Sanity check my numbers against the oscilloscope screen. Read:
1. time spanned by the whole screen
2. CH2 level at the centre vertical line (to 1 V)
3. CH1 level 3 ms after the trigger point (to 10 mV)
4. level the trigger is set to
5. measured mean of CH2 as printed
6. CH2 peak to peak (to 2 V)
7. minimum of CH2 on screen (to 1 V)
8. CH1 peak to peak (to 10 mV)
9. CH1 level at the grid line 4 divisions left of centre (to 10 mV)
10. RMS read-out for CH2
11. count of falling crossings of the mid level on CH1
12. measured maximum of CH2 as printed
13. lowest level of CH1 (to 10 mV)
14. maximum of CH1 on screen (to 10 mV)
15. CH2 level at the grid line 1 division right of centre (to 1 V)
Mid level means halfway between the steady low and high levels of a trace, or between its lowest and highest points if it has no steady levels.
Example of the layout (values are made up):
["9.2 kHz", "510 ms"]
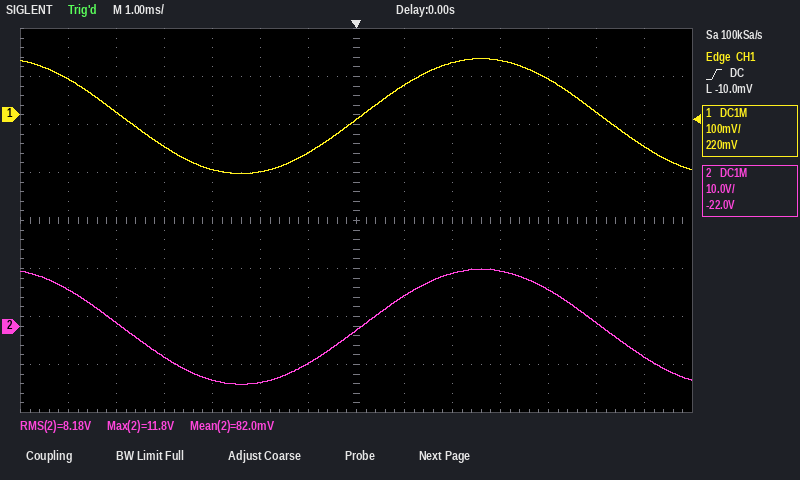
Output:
["14 ms", "-1 V", "110 mV", "-10.0 mV", "82.0 mV", "24 V", "-12 V", "240 mV", "-70 mV", "8.18 V", "2", "11.8 V", "-120 mV", "120 mV", "6 V"]
